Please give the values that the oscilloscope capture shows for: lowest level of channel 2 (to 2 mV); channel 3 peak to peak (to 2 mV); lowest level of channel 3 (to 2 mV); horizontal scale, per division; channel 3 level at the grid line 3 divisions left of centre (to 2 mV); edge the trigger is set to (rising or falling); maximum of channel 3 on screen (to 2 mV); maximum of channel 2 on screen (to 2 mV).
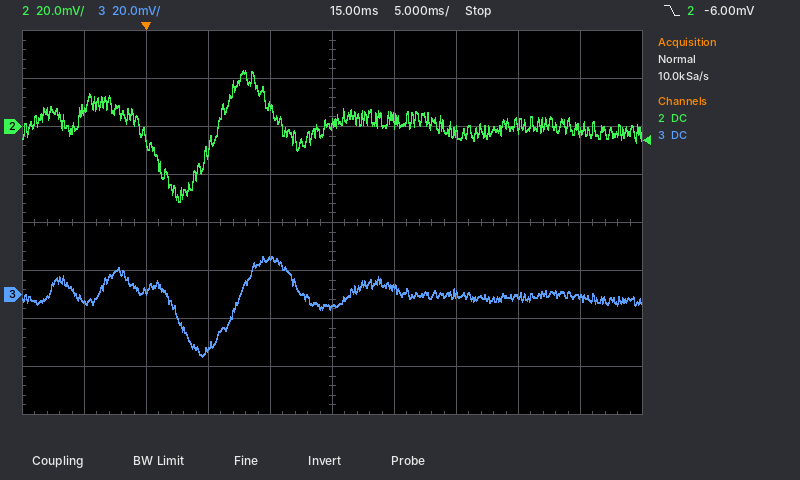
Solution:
-32 mV
42 mV
-26 mV
5 ms
2 mV
falling
16 mV
24 mV
